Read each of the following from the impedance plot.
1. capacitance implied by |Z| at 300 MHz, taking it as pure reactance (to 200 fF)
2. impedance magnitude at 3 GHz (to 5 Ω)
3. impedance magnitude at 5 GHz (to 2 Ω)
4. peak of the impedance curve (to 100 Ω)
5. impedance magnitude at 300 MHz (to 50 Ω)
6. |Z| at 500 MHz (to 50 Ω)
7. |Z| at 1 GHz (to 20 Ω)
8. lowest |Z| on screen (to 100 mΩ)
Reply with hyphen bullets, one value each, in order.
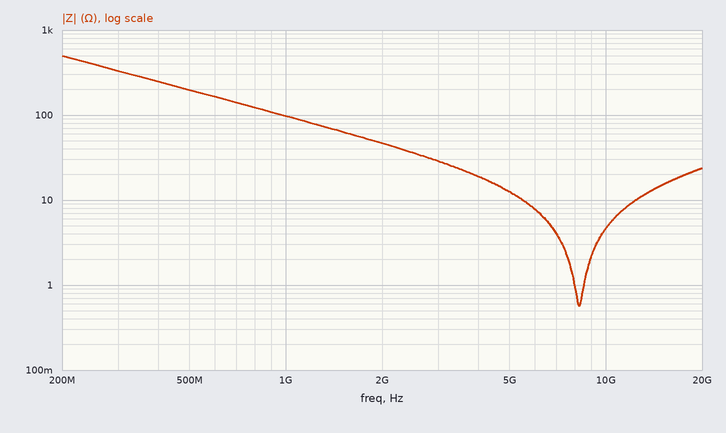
- 1.6 pF
- 30 Ω
- 12 Ω
- 500 Ω
- 350 Ω
- 200 Ω
- 100 Ω
- 600 mΩ
